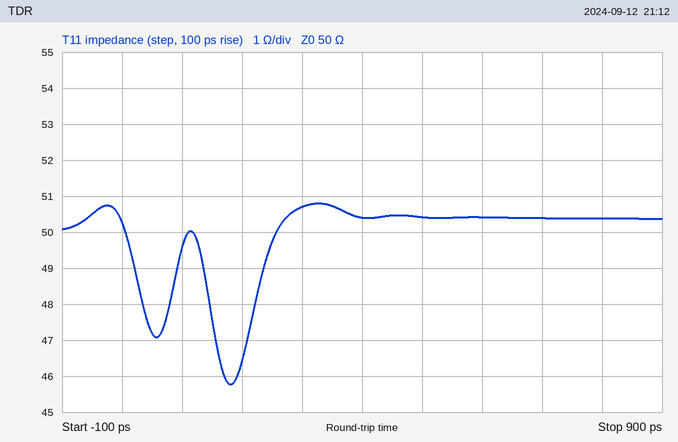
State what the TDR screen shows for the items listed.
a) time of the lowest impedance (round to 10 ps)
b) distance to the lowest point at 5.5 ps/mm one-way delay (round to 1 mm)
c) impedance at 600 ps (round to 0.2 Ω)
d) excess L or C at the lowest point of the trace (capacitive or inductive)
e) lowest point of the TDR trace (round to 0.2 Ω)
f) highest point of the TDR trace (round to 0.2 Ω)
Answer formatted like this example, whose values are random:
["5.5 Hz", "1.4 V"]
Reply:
["180 ps", "16 mm", "50.4 Ω", "capacitive", "45.8 Ω", "50.8 Ω"]
